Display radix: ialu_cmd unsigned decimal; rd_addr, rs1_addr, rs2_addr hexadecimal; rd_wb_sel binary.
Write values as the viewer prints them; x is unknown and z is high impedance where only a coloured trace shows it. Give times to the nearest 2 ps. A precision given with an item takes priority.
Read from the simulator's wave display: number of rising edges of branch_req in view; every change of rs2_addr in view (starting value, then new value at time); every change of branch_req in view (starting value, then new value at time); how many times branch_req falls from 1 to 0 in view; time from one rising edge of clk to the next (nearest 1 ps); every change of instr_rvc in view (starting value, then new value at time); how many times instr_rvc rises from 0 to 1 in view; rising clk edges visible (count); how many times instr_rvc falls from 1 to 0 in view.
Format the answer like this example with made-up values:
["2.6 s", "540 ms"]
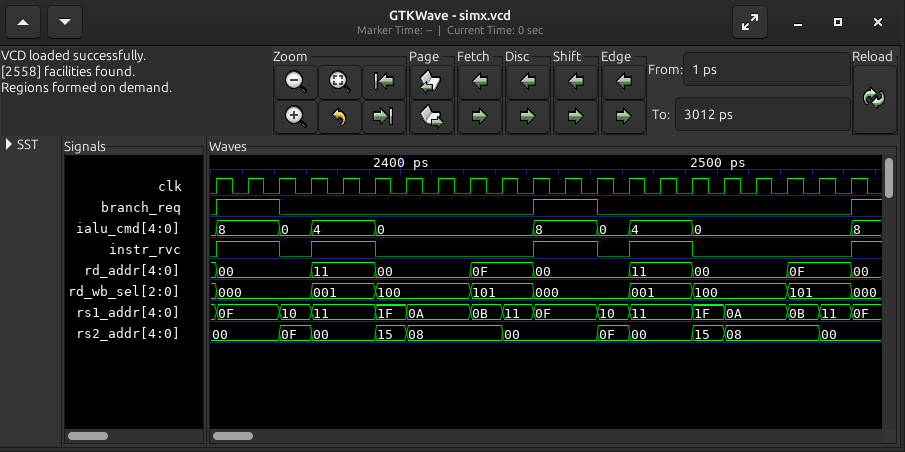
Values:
["3", "00, 0F at 2362 ps, 00 at 2372 ps, 15 at 2392 ps, 08 at 2402 ps, 00 at 2432 ps, 0F at 2462 ps, 00 at 2472 ps, 15 at 2492 ps, 08 at 2502 ps, 00 at 2532 ps", "0, 1 at 2342 ps, 0 at 2362 ps, 1 at 2442 ps, 0 at 2462 ps, 1 at 2542 ps", "2", "10 ps", "0, 1 at 2342 ps, 0 at 2362 ps, 1 at 2372 ps, 0 at 2392 ps, 1 at 2442 ps, 0 at 2462 ps, 1 at 2472 ps, 0 at 2492 ps, 1 at 2542 ps", "5", "21", "4"]
